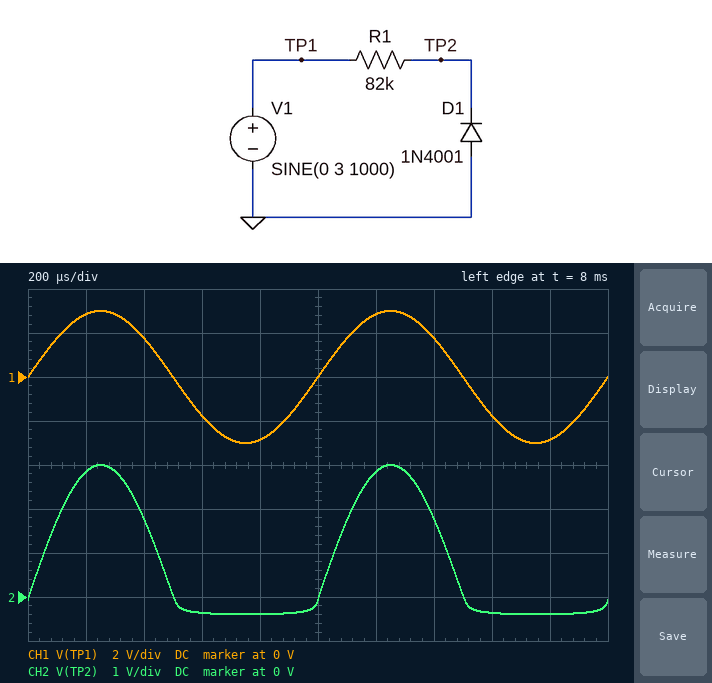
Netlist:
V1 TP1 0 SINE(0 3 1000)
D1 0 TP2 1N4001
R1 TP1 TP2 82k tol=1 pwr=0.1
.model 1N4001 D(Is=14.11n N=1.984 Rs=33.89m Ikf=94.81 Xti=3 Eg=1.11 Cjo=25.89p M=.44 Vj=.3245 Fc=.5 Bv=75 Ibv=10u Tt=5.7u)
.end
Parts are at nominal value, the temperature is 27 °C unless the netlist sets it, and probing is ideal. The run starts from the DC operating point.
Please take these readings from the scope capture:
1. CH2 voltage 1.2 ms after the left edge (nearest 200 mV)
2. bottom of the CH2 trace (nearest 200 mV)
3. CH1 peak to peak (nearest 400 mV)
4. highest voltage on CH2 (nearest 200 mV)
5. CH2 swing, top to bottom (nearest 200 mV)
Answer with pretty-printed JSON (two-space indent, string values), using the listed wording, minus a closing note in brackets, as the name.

{
  "CH2 voltage 1.2 ms after the left edge": "2.8 V",
  "bottom of the CH2 trace": "-400 mV",
  "CH1 peak to peak": "6.0 V",
  "highest voltage on CH2": "3.0 V",
  "CH2 swing, top to bottom": "3.4 V"
}
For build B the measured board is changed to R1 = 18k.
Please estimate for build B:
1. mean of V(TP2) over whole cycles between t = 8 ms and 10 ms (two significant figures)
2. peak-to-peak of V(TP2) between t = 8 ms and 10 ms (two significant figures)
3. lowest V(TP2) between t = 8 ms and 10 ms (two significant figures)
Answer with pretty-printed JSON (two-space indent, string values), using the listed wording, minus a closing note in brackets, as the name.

{
  "mean of V(TP2) over whole cycles between t = 8 ms and 10 ms": "750 mV",
  "peak-to-peak of V(TP2) between t = 8 ms and 10 ms": "3.5 V",
  "lowest V(TP2) between t = 8 ms and 10 ms": "-470 mV"
}
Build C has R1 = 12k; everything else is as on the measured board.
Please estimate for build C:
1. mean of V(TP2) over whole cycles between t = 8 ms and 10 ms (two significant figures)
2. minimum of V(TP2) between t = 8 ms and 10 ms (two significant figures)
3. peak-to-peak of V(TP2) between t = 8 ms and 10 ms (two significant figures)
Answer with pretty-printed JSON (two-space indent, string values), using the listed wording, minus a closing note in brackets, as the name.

{
  "mean of V(TP2) over whole cycles between t = 8 ms and 10 ms": "740 mV",
  "minimum of V(TP2) between t = 8 ms and 10 ms": "-490 mV",
  "peak-to-peak of V(TP2) between t = 8 ms and 10 ms": "3.5 V"
}
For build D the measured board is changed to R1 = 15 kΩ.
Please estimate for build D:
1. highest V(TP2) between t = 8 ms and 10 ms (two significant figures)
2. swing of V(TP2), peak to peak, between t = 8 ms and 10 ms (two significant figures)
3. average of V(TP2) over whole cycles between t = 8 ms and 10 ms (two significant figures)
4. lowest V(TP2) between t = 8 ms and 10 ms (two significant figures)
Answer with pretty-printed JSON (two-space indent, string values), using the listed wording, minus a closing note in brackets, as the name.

{
  "highest V(TP2) between t = 8 ms and 10 ms": "3.0 V",
  "swing of V(TP2), peak to peak, between t = 8 ms and 10 ms": "3.5 V",
  "average of V(TP2) over whole cycles between t = 8 ms and 10 ms": "740 mV",
  "lowest V(TP2) between t = 8 ms and 10 ms": "-480 mV"
}
